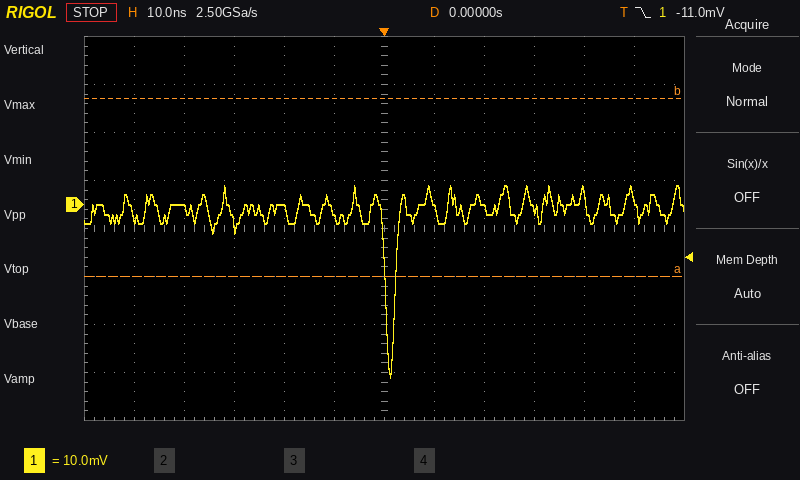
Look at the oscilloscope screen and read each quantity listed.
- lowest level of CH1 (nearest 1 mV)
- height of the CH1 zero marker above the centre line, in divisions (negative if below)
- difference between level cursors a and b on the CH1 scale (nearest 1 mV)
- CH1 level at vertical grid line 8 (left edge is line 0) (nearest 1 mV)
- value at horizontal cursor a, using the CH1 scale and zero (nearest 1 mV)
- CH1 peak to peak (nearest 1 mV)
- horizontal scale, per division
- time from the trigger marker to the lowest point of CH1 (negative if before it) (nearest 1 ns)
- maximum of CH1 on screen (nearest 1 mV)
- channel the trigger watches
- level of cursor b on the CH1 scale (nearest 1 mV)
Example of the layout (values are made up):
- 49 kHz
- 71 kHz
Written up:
- -36 mV
- +0.5 div
- 37 mV
- -1 mV
- -15 mV
- 40 mV
- 10 ns
- +1 ns
- 4 mV
- CH1
- 22 mV
